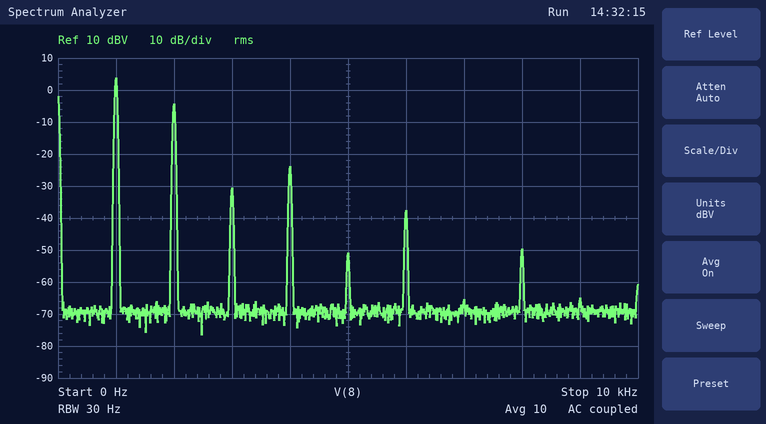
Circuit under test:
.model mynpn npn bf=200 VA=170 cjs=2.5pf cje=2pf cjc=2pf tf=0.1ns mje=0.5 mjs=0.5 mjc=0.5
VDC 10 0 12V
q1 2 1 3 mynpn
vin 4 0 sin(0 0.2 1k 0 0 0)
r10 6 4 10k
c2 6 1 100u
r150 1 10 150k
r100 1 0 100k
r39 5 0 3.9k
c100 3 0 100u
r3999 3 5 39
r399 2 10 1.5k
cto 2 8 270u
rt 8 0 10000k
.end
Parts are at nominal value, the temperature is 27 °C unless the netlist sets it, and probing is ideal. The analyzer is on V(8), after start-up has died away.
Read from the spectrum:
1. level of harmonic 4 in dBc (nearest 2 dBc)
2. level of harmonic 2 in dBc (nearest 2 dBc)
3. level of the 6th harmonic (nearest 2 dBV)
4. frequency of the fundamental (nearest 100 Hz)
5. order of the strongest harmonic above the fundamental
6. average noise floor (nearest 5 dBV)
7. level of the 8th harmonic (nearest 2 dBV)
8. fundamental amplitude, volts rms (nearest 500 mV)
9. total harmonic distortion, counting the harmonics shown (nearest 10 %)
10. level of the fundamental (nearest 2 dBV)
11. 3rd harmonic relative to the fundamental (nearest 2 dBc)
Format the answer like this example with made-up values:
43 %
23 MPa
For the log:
-28 dBc
-8 dBc
-38 dBV
1.0 kHz
2
-70 dBV
-50 dBV
1.5 V
40 %
4 dBV
-34 dBc
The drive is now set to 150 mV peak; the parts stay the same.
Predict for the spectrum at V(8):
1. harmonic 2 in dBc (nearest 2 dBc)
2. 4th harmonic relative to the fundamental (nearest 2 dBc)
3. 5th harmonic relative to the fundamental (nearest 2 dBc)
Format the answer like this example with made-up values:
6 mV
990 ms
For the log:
-10 dBc
-34 dBc
-46 dBc
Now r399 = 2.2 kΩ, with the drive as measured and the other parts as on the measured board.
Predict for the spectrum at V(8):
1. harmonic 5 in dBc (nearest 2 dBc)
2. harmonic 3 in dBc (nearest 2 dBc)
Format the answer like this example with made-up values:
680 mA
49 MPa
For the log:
-58 dBc
-36 dBc
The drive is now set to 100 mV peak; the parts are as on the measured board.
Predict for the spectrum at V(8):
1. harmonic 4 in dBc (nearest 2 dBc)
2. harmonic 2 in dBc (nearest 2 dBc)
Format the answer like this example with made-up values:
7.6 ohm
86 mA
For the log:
-52 dBc
-16 dBc
